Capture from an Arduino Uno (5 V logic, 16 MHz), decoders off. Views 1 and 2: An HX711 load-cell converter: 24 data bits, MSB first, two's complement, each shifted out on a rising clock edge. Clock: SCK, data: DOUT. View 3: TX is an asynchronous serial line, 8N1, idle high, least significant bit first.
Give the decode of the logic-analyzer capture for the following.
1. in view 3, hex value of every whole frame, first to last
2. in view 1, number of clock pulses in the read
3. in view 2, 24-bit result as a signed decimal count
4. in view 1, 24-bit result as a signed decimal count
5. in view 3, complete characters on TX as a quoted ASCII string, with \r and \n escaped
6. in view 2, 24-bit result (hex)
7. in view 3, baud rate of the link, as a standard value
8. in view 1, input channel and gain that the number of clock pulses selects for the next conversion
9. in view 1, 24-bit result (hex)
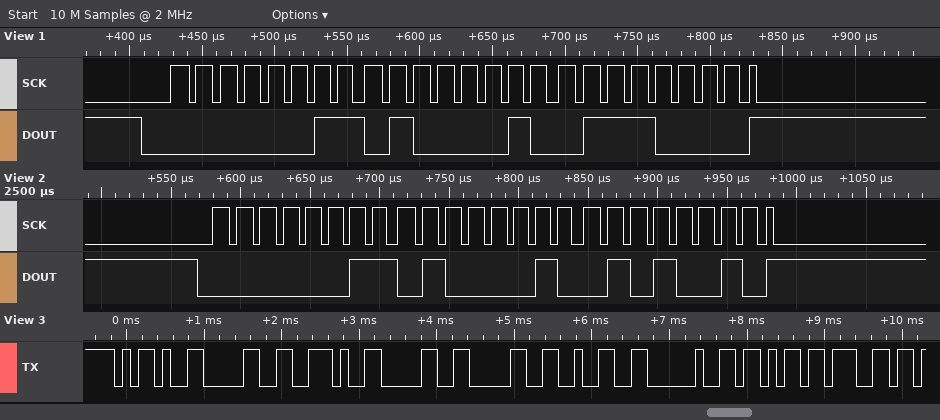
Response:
0x2D 0x30 0x2E 0x30 0x30 0x32 0x20 0x6B 0x67
25
213586
213616
"-0.002 kg"
0x034252
9600 baud
channel A, gain 128
0x034270
